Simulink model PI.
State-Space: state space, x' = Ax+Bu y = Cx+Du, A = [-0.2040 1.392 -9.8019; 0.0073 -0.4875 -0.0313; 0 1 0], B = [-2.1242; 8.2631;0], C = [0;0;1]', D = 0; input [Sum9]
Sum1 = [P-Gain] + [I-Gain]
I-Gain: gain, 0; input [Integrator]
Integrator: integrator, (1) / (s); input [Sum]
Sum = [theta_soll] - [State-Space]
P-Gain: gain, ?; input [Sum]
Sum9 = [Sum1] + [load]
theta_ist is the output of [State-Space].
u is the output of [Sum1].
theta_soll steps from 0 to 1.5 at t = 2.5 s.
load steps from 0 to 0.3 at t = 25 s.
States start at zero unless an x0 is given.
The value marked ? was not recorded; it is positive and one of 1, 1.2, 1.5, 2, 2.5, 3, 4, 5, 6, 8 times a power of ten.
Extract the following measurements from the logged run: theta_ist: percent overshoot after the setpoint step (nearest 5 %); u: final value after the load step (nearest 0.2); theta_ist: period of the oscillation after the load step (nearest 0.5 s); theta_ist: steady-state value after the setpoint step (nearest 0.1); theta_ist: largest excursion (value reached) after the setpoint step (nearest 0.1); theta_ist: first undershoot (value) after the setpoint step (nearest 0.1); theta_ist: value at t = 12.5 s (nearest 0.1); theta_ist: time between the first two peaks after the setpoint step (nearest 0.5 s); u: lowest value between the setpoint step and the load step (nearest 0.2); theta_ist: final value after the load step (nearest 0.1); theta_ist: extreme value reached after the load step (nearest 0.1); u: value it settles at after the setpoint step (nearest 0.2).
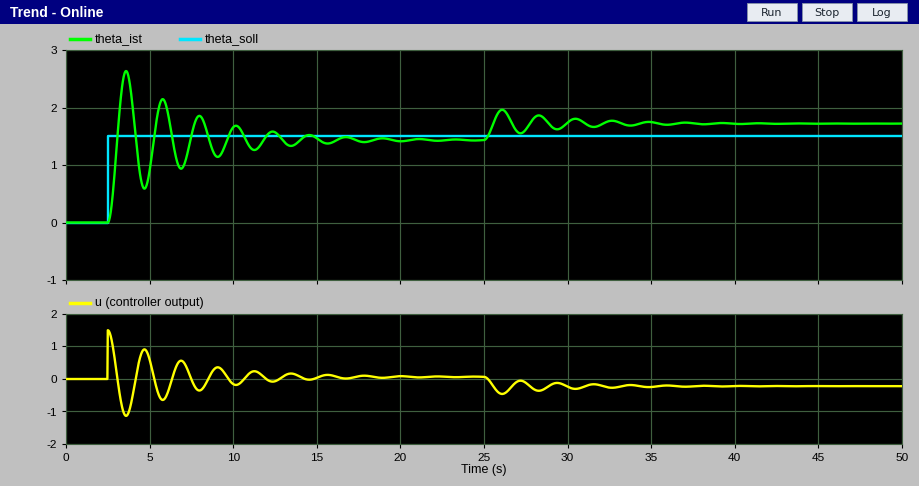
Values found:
85 %
-0.2
2.0 s
1.4
2.6
0.6
1.6
2.0 s
-1.2
1.7
2.0
0.0
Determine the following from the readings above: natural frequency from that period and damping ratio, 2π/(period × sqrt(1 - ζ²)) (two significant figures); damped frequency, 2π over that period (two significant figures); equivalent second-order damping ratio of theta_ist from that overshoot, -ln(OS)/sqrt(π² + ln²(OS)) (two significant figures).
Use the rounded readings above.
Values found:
3.1 rad/s
3.1 rad/s
0.052
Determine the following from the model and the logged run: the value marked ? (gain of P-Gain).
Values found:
1
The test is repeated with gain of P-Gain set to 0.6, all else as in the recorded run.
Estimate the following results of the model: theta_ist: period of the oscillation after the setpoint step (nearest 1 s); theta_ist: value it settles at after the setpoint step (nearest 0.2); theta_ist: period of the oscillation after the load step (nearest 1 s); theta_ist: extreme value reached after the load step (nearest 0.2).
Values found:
3 s
1.4
3 s
2.2
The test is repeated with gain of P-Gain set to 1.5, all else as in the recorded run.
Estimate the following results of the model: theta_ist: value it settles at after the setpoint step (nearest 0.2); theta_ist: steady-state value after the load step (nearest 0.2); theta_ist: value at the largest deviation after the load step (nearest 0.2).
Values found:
1.4
1.6
1.8
